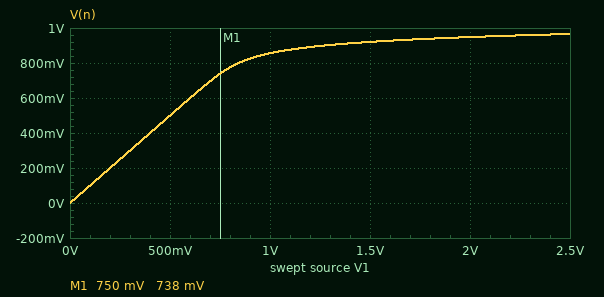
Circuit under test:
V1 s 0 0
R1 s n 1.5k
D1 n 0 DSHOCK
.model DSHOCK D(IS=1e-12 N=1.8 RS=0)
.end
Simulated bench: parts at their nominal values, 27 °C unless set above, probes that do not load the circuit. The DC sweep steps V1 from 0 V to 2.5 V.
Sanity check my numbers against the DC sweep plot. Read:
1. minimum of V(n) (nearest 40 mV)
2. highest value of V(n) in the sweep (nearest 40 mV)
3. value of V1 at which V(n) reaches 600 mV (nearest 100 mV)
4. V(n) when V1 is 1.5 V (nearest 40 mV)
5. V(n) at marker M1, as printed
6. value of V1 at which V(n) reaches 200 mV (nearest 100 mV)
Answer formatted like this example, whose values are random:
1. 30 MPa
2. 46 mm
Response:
1. 0 V
2. 960 mV
3. 600 mV
4. 920 mV
5. 738 mV
6. 200 mV
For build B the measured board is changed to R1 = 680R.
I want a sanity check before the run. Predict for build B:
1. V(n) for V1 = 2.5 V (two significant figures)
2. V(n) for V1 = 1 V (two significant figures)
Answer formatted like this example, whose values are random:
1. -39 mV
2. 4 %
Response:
1. 1.0 V
2. 880 mV
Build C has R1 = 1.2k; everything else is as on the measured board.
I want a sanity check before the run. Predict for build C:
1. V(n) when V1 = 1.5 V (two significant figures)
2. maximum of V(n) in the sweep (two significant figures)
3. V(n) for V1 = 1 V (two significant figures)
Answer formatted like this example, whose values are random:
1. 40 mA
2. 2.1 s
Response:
1. 930 mV
2. 980 mV
3. 860 mV
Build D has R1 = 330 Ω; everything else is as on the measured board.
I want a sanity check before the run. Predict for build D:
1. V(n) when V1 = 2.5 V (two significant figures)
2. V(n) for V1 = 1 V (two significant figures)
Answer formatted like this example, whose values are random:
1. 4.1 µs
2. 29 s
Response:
1. 1.0 V
2. 910 mV
